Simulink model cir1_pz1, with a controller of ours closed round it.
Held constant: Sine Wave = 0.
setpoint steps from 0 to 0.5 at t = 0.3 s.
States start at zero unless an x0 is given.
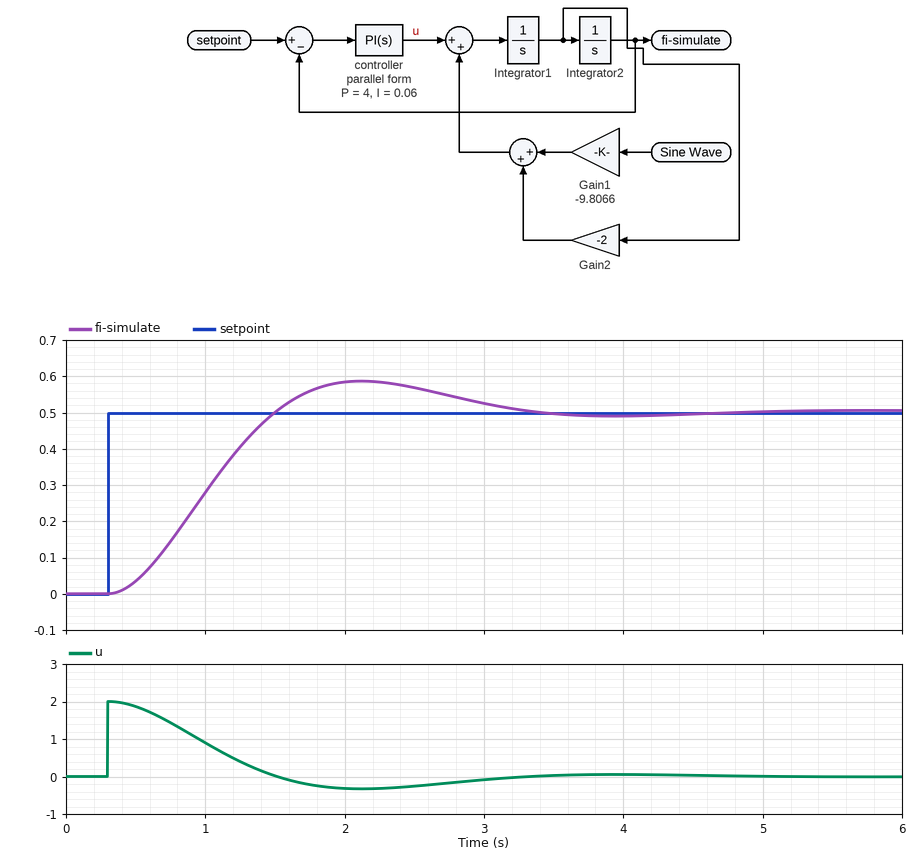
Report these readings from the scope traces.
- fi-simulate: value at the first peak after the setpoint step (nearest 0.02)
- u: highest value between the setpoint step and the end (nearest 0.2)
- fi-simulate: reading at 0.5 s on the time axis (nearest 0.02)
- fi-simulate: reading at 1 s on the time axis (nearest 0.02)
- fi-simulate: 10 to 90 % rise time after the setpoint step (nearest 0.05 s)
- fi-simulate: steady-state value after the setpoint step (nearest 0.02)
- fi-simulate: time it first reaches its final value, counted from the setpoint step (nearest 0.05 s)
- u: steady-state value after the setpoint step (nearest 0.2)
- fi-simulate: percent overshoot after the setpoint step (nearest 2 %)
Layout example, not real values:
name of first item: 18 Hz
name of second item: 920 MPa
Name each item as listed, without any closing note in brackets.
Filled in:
fi-simulate: value at the first peak after the setpoint step: 0.58
u: highest value between the setpoint step and the end: 2.0
fi-simulate: reading at 0.5 s on the time axis: 0.04
fi-simulate: reading at 1 s on the time axis: 0.28
fi-simulate: 10 to 90 % rise time after the setpoint step: 0.80 s
fi-simulate: steady-state value after the setpoint step: 0.50
fi-simulate: time it first reaches its final value, counted from the setpoint step: 1.20 s
u: steady-state value after the setpoint step: 0.0
fi-simulate: percent overshoot after the setpoint step: 16 %
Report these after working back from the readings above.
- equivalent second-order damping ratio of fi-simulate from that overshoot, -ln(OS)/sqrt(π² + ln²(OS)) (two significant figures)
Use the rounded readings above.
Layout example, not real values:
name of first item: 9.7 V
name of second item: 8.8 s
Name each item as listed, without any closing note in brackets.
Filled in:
equivalent second-order damping ratio of fi-simulate from that overshoot, -ln(OS)/sqrt(π² + ln²(OS)): 0.50
